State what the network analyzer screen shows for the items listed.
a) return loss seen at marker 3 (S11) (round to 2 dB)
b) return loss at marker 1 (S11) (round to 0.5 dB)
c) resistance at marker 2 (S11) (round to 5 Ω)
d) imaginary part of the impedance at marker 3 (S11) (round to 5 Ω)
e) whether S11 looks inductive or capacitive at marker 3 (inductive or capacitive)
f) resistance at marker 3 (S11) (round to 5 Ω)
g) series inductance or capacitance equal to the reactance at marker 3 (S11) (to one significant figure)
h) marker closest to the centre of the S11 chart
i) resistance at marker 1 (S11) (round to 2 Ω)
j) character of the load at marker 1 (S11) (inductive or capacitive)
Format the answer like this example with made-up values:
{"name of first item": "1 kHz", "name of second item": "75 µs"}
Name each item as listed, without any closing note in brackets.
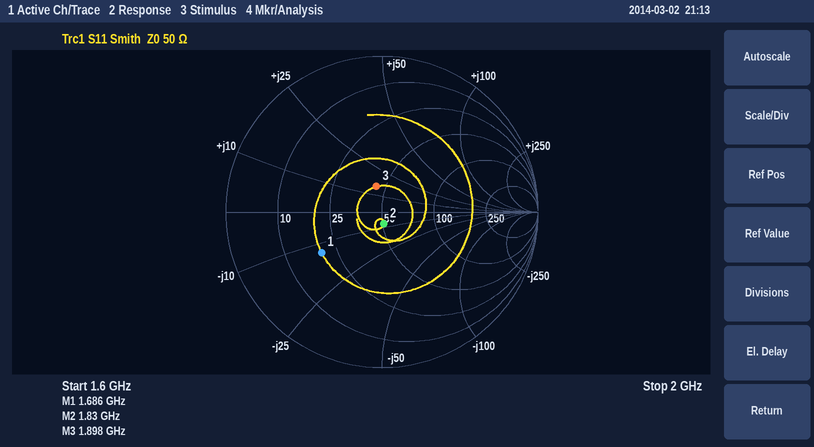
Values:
{"return loss seen at marker 3 (S11)": "16 dB", "return loss at marker 1 (S11)": "6.5 dB", "resistance at marker 2 (S11)": "50 Ω", "imaginary part of the impedance at marker 3 (S11)": "+15 Ω", "whether S11 looks inductive or capacitive at marker 3": "inductive", "resistance at marker 3 (S11)": "45 Ω", "series inductance or capacitance equal to the reactance at marker 3 (S11)": "1 nH", "marker closest to the centre of the S11 chart": "marker 2", "resistance at marker 1 (S11)": "20 Ω", "character of the load at marker 1 (S11)": "capacitive"}
